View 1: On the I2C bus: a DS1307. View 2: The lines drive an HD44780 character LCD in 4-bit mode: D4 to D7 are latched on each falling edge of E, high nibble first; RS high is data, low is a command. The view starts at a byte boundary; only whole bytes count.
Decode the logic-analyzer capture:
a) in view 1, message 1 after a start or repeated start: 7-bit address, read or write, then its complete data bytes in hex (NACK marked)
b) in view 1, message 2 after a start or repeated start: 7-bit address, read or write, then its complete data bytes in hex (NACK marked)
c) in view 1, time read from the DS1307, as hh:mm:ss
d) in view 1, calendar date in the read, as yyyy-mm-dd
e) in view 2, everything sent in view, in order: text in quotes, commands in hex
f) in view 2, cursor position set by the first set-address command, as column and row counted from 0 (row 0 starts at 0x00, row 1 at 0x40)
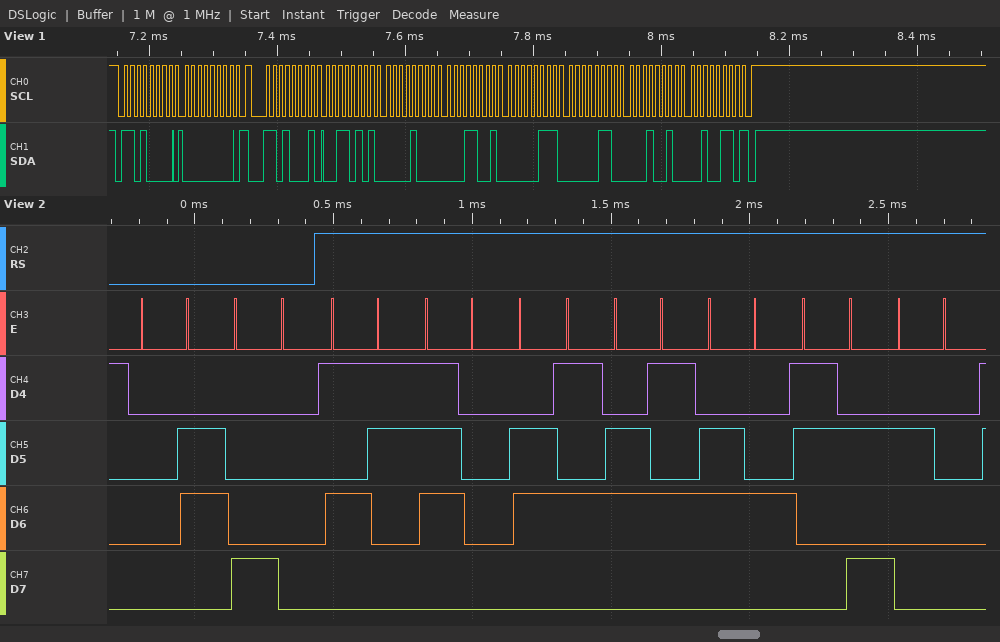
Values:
0x68 write: 00
0x68 read: 35 08 19 07 06 12 26 NACK
19:08:35
2026-12-06
0x06 0x80 "Speed: "
column 0, row 0
